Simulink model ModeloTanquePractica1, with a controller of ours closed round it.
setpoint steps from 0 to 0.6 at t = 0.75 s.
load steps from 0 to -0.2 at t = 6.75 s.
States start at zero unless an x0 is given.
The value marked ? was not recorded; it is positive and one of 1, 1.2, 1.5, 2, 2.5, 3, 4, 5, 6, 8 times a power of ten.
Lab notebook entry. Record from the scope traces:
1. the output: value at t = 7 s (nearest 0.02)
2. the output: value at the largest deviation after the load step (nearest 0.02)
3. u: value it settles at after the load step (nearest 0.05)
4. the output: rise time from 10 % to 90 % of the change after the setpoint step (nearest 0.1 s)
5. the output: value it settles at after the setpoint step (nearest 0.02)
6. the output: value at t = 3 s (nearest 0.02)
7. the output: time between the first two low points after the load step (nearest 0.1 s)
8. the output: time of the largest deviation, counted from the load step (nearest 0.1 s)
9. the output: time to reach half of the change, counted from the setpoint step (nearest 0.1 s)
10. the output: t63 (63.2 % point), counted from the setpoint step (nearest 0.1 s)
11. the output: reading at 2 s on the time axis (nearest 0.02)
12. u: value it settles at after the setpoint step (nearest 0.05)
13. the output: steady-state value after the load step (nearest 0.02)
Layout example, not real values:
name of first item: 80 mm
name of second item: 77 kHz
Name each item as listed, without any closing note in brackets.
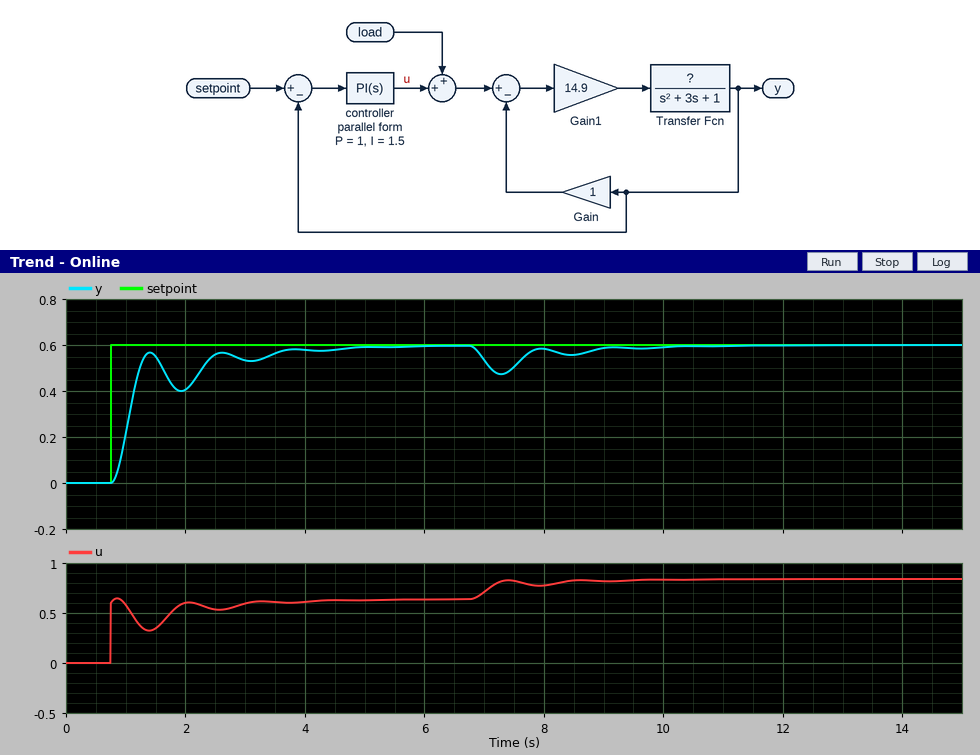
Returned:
the output: value at t = 7 s: 0.54
the output: value at the largest deviation after the load step: 0.48
u: value it settles at after the load step: 0.85
the output: rise time from 10 % to 90 % of the change after the setpoint step: 0.4 s
the output: value it settles at after the setpoint step: 0.60
the output: value at t = 3 s: 0.54
the output: time between the first two low points after the load step: 1.2 s
the output: time of the largest deviation, counted from the load step: 0.5 s
the output: time to reach half of the change, counted from the setpoint step: 0.3 s
the output: t63 (63.2 % point), counted from the setpoint step: 0.4 s
the output: reading at 2 s on the time axis: 0.40
u: value it settles at after the setpoint step: 0.65
the output: steady-state value after the load step: 0.60
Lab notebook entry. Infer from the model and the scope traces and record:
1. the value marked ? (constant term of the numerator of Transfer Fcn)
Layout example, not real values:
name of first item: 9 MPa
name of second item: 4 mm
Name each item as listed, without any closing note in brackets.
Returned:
the value marked ?: 1
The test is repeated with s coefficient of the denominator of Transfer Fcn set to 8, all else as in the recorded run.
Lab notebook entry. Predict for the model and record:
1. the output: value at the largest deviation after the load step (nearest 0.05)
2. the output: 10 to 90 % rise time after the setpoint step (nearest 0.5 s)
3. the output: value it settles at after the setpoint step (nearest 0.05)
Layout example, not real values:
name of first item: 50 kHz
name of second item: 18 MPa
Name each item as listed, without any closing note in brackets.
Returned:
the output: value at the largest deviation after the load step: 0.50
the output: 10 to 90 % rise time after the setpoint step: 1.5 s
the output: value it settles at after the setpoint step: 0.60
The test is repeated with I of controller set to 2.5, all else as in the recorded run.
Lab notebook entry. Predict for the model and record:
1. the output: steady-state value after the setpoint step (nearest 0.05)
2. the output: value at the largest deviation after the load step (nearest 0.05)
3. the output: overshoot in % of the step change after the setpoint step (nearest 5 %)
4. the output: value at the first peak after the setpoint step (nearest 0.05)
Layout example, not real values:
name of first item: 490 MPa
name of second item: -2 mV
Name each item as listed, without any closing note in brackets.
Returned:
the output: steady-state value after the setpoint step: 0.60
the output: value at the largest deviation after the load step: 0.50
the output: overshoot in % of the step change after the setpoint step: 10 %
the output: value at the first peak after the setpoint step: 0.65
